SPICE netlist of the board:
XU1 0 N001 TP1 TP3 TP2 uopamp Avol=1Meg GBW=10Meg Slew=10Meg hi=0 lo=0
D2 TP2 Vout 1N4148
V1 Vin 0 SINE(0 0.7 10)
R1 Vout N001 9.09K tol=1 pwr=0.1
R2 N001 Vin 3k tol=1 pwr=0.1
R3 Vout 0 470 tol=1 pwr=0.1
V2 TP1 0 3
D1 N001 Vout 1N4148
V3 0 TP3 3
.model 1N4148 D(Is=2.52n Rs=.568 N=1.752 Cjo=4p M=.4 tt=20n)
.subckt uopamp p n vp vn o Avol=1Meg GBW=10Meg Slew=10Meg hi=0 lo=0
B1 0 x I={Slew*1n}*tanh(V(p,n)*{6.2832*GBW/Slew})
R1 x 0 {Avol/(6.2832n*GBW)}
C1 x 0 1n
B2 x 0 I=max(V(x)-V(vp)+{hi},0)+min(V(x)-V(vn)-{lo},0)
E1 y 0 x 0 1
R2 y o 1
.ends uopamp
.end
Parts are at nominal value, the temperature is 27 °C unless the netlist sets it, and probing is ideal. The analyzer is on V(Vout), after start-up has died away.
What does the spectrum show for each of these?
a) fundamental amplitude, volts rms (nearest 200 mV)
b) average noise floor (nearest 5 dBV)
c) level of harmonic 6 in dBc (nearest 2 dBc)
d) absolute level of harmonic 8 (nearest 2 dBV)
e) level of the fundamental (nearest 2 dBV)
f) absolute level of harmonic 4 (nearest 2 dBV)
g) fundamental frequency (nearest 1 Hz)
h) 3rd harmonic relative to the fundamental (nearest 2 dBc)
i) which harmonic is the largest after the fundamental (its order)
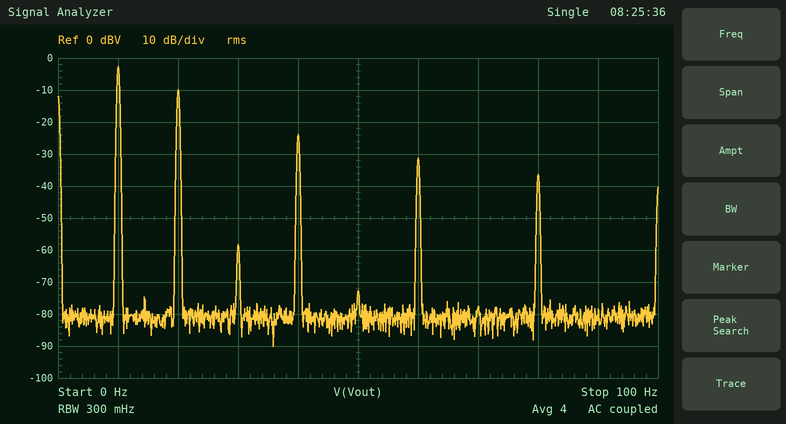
800 mV
-80 dBV
-28 dBc
-36 dBV
-2 dBV
-24 dBV
10 Hz
-56 dBc
2
